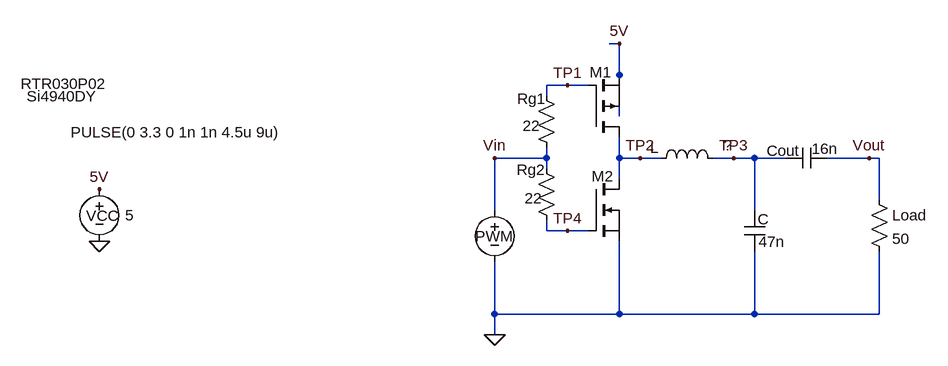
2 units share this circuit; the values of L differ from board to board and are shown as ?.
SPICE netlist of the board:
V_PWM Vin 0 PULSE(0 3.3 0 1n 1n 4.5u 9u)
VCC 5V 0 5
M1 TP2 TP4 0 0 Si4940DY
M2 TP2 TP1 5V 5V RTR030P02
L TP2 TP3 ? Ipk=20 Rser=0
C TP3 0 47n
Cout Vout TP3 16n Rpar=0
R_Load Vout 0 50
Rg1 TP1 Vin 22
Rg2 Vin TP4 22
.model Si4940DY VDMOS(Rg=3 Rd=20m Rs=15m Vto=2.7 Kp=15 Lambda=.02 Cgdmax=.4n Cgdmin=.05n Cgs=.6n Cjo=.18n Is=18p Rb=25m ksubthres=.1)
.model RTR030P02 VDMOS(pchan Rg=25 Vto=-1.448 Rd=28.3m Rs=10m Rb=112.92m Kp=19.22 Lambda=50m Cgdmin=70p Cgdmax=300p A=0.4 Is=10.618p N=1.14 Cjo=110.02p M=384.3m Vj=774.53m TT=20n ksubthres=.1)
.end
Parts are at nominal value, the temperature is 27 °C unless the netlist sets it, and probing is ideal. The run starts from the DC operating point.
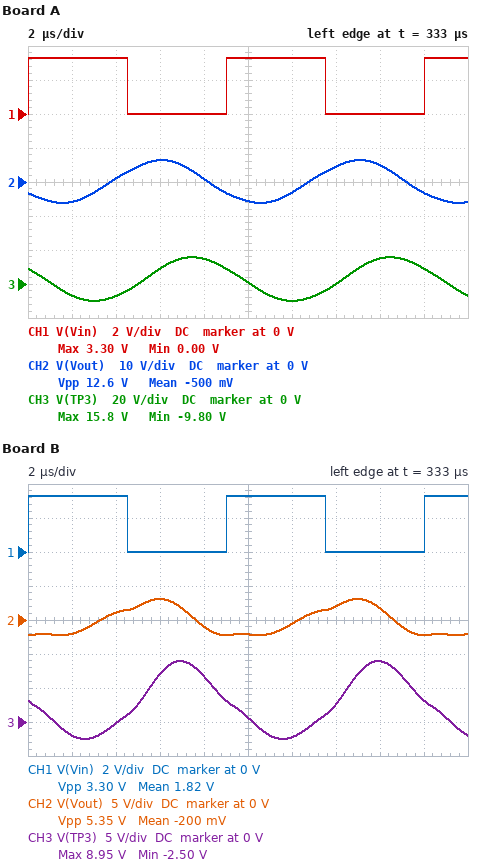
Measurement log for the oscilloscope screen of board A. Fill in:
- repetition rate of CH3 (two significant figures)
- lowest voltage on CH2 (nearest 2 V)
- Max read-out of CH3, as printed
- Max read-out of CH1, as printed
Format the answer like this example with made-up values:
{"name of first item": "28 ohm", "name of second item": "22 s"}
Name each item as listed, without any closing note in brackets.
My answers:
{"repetition rate of CH3": "110 kHz", "lowest voltage on CH2": "-6 V", "Max read-out of CH3, as printed": "15.8 V", "Max read-out of CH1, as printed": "3.30 V"}
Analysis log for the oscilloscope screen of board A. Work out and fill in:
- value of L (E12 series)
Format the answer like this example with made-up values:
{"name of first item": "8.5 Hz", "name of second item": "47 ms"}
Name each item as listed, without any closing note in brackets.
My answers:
{"value of L": "27 µH"}
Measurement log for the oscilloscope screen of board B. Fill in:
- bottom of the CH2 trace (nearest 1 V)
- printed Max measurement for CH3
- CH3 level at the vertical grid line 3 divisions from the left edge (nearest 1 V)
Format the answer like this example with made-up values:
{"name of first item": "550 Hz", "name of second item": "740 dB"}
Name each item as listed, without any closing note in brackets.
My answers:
{"bottom of the CH2 trace": "-2 V", "printed Max measurement for CH3": "8.95 V", "CH3 level at the vertical grid line 3 divisions from the left edge": "7 V"}
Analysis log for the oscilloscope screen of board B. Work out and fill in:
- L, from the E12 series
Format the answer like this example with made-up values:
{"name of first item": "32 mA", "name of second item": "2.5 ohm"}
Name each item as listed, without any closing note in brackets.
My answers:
{"L, from the E12 series": "15 µH"}
